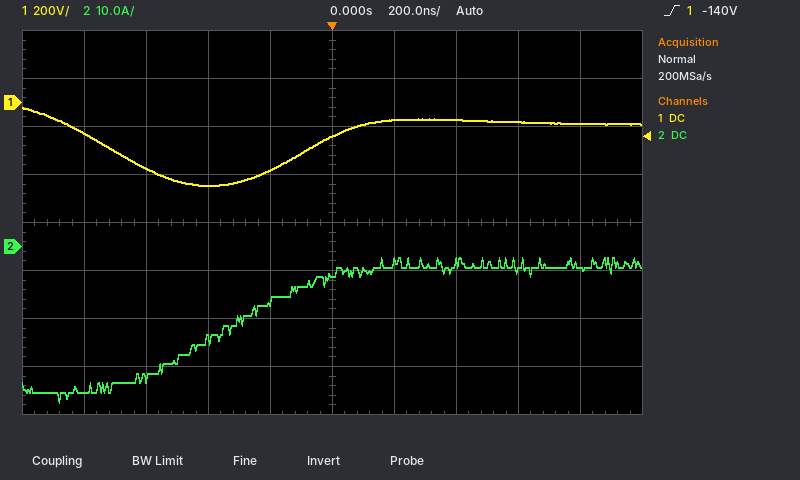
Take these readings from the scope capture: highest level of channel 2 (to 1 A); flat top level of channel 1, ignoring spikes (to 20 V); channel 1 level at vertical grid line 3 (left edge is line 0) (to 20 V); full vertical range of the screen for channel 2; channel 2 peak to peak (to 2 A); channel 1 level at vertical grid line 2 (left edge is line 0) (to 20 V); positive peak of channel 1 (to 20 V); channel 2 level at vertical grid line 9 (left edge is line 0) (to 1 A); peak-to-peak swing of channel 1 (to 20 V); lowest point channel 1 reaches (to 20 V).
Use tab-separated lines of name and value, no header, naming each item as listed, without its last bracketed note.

highest level of channel 2	-2 A
flat top level of channel 1, ignoring spikes	-80 V
channel 1 level at vertical grid line 3 (left edge is line 0)	-340 V
full vertical range of the screen for channel 2	80 A
channel 2 peak to peak	30 A
channel 1 level at vertical grid line 2 (left edge is line 0)	-280 V
positive peak of channel 1	-20 V
channel 2 level at vertical grid line 9 (left edge is line 0)	-5 A
peak-to-peak swing of channel 1	320 V
lowest point channel 1 reaches	-340 V
